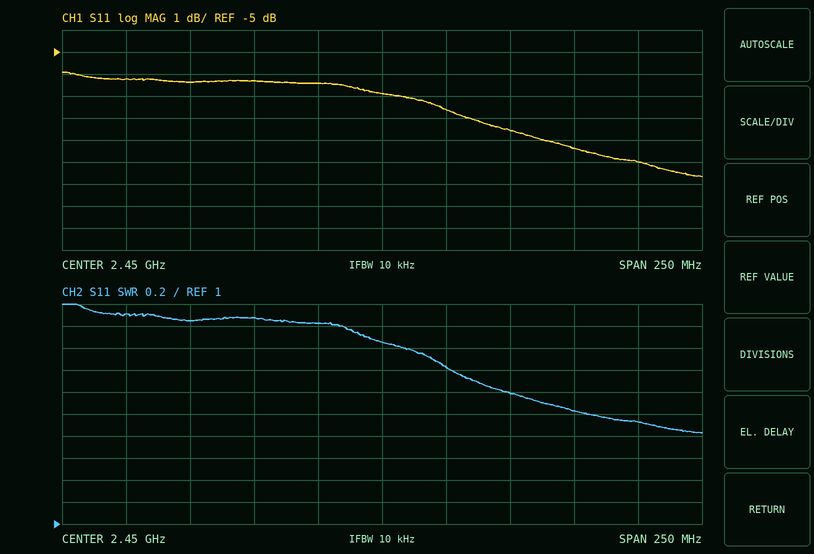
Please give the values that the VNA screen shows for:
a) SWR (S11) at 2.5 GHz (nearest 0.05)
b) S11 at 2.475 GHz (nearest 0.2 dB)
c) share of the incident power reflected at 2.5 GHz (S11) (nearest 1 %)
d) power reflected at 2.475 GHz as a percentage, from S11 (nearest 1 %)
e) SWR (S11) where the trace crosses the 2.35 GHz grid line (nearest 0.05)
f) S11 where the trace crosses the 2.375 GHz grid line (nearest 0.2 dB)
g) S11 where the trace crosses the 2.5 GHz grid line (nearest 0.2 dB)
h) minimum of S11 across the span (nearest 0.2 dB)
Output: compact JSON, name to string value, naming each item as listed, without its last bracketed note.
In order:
{"SWR (S11) at 2.5 GHz": "2.20", "S11 at 2.475 GHz": "-7.6 dB", "share of the incident power reflected at 2.5 GHz (S11)": "14 %", "power reflected at 2.475 GHz as a percentage, from S11": "17 %", "SWR (S11) where the trace crosses the 2.35 GHz grid line": "2.90", "S11 where the trace crosses the 2.375 GHz grid line": "-6.4 dB", "S11 where the trace crosses the 2.5 GHz grid line": "-8.6 dB", "minimum of S11 across the span": "-10.6 dB"}
